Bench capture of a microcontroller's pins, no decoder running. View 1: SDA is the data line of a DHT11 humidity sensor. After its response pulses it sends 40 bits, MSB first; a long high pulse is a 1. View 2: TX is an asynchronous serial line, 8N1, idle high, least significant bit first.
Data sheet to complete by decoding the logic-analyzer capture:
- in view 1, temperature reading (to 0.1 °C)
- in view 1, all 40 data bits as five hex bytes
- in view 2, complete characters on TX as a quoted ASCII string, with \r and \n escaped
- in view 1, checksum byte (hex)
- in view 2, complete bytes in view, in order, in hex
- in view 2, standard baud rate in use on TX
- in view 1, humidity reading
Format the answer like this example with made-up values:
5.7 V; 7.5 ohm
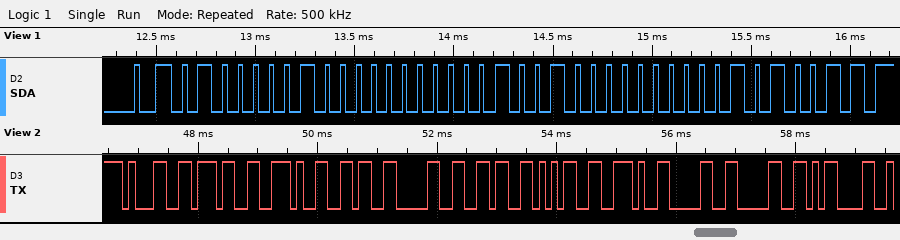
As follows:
18.0 °C; 41 00 12 00 53; "17.6065.00\r"; 0x53; 31 37 2E 36 30 36 35 2E 30 30 0D; 9600 baud; 65 %
